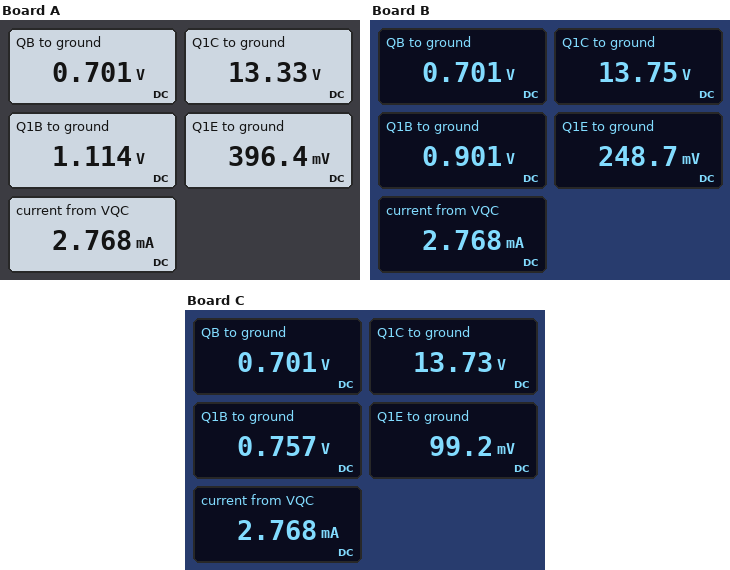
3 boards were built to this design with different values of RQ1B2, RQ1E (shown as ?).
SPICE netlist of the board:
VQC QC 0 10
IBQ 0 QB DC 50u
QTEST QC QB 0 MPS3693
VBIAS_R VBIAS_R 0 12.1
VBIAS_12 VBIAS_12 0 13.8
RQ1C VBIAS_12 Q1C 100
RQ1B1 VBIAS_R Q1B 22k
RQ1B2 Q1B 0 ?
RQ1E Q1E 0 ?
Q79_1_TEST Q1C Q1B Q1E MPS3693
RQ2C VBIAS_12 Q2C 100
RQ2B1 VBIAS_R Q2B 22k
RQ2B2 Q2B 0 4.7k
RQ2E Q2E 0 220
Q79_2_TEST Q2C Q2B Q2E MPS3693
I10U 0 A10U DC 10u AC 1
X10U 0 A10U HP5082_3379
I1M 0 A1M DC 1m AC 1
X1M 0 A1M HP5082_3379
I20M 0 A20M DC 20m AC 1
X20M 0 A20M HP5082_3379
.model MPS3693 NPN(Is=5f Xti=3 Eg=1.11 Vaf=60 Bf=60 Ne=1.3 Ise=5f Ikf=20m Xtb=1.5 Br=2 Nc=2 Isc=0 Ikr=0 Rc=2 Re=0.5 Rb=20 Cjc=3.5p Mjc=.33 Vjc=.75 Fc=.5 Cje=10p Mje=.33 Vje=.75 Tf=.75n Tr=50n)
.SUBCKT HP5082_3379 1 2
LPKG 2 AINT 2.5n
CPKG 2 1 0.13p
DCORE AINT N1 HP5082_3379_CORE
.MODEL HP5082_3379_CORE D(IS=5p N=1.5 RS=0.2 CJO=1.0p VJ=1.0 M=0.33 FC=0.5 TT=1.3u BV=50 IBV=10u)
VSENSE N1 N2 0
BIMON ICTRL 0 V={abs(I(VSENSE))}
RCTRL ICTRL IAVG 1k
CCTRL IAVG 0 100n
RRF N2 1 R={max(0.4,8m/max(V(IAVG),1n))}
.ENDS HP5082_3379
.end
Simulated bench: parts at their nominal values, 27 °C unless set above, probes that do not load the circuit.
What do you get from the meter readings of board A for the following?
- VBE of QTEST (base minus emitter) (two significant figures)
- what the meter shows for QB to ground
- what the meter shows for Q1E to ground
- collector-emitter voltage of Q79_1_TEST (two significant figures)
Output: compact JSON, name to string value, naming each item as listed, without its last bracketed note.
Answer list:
{"VBE of QTEST (base minus emitter)": "700 mV", "what the meter shows for QB to ground": "0.701 V", "what the meter shows for Q1E to ground": "396.4 mV", "collector-emitter voltage of Q79_1_TEST": "13 V"}
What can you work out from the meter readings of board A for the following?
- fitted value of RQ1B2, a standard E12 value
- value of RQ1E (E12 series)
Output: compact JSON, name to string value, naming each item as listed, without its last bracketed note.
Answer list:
{"fitted value of RQ1B2, a standard E12 value": "2.7 kΩ", "value of RQ1E": "82 Ω"}
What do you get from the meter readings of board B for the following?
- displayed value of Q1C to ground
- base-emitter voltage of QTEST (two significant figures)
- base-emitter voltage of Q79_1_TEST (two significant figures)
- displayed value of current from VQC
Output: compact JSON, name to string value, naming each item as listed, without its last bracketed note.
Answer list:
{"displayed value of Q1C to ground": "13.75 V", "base-emitter voltage of QTEST": "700 mV", "base-emitter voltage of Q79_1_TEST": "650 mV", "displayed value of current from VQC": "2.768 mA"}
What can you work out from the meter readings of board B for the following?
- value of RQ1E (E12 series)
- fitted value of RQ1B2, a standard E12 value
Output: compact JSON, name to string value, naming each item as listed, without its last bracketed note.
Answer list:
{"value of RQ1E": "470 Ω", "fitted value of RQ1B2, a standard E12 value": "1.8 kΩ"}
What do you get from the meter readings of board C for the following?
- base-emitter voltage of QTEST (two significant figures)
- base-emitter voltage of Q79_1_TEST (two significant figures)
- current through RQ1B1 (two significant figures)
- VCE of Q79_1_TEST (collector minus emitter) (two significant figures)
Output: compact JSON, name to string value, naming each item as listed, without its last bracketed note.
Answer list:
{"base-emitter voltage of QTEST": "700 mV", "base-emitter voltage of Q79_1_TEST": "660 mV", "current through RQ1B1": "520 µA", "VCE of Q79_1_TEST (collector minus emitter)": "14 V"}
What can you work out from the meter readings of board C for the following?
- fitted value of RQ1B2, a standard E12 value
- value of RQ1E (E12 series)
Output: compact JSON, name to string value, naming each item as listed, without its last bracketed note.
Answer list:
{"fitted value of RQ1B2, a standard E12 value": "1.5 kΩ", "value of RQ1E": "150 Ω"}
